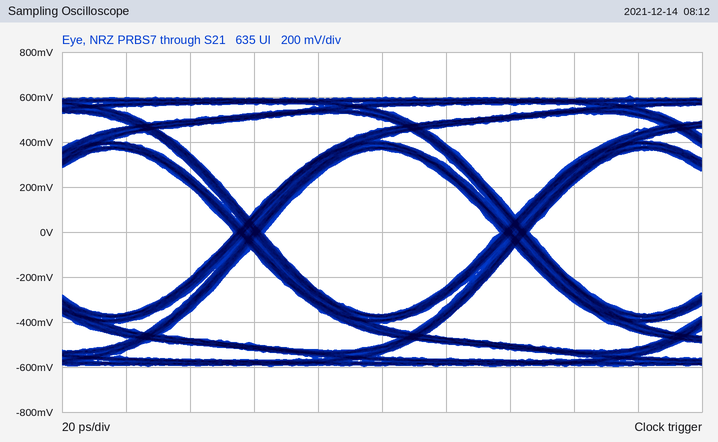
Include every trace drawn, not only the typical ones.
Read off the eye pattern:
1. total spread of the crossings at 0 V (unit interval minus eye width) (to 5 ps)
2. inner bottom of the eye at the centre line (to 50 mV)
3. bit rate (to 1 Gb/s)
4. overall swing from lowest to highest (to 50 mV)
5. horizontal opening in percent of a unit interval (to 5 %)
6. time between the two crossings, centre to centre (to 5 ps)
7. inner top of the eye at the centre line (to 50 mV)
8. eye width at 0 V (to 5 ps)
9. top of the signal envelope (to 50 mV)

10 ps
-350 mV
12 Gb/s
1.20 V
90 %
85 ps
350 mV
75 ps
600 mV
